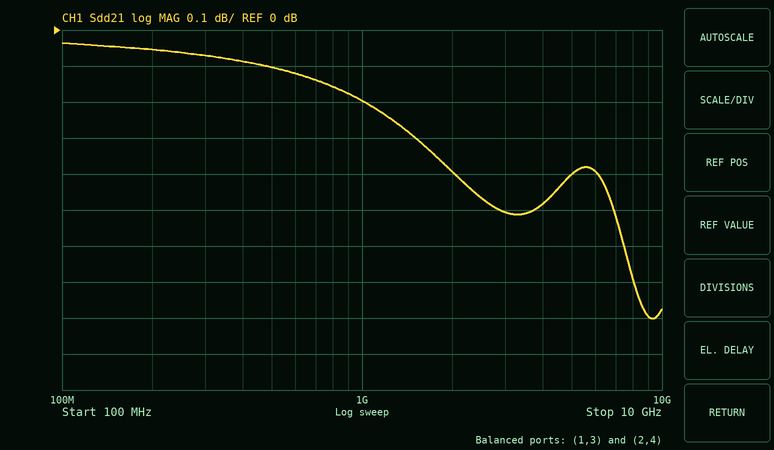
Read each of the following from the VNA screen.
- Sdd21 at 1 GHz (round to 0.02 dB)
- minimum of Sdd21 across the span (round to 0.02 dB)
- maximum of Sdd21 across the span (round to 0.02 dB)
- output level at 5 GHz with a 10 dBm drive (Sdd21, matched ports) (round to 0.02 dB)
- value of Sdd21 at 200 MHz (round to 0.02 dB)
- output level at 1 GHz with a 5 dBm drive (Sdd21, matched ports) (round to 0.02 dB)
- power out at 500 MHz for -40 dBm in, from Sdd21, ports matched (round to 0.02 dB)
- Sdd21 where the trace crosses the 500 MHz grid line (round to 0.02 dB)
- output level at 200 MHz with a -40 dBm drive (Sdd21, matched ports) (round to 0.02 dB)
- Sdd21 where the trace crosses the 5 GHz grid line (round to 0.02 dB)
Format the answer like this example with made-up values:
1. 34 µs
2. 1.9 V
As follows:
1. -0.20 dB
2. -0.80 dB
3. -0.04 dB
4. 9.60 dBm
5. -0.06 dB
6. 4.80 dBm
7. -40.10 dBm
8. -0.10 dB
9. -40.06 dBm
10. -0.40 dB
